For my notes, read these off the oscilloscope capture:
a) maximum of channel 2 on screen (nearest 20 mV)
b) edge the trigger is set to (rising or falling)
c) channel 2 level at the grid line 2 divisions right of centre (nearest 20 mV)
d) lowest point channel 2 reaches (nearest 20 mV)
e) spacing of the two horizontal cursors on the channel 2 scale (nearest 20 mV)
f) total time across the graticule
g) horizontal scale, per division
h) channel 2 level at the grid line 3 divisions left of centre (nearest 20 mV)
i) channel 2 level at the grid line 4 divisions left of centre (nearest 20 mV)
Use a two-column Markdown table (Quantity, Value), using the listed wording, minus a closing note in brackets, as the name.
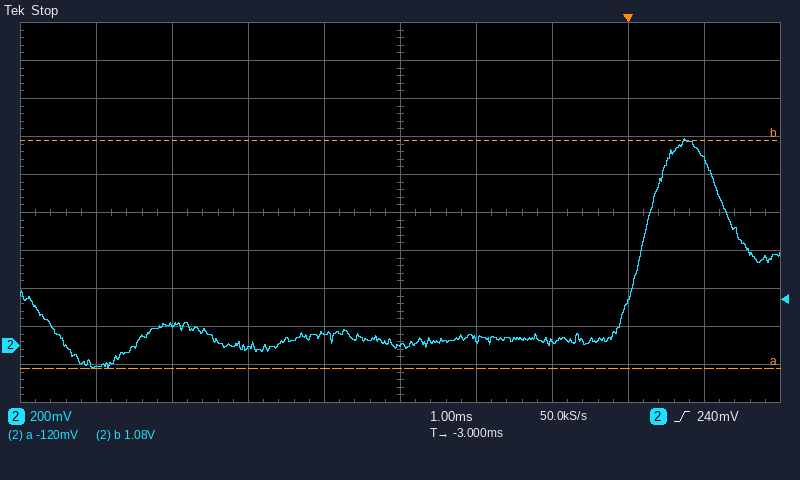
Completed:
| Quantity | Value |
|---|---|
| maximum of channel 2 on screen | 1.08 V |
| edge the trigger is set to | rising |
| channel 2 level at the grid line 2 divisions right of centre | 20 mV |
| lowest point channel 2 reaches | -120 mV |
| spacing of the two horizontal cursors on the channel 2 scale | 1.20 V |
| total time across the graticule | 10 ms |
| horizontal scale, per division | 1 ms |
| channel 2 level at the grid line 3 divisions left of centre | 100 mV |
| channel 2 level at the grid line 4 divisions left of centre | -120 mV |
